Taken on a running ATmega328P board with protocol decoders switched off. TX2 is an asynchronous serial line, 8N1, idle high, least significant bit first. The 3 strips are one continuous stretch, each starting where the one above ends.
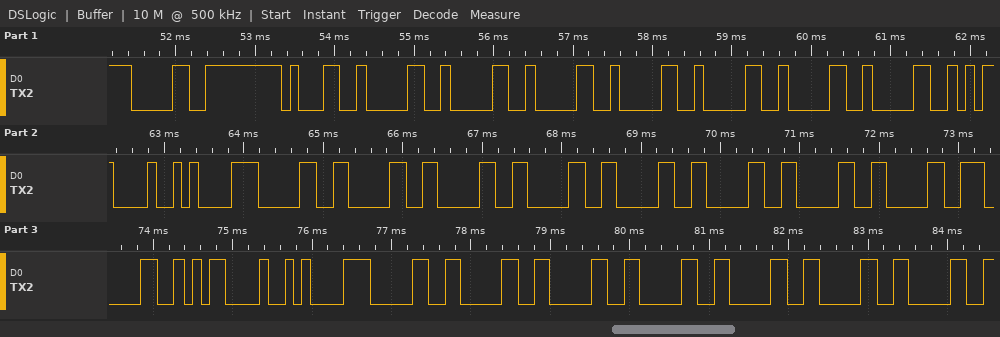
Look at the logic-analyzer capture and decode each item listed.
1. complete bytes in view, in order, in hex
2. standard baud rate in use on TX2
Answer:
30 31 30 30 30 30 30 30 30 0D 0A 30 30 30 30 30 30 30 30 30 0D 0A 30 30 30 30 30 30 30
9600 baud
